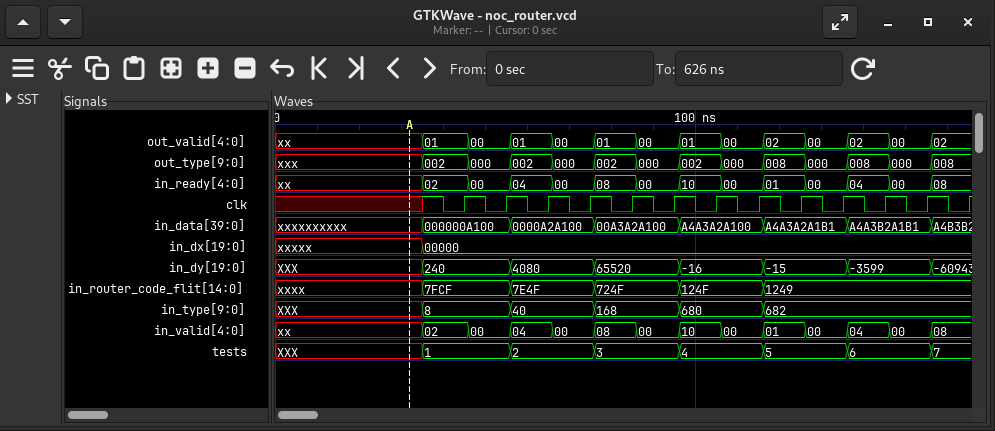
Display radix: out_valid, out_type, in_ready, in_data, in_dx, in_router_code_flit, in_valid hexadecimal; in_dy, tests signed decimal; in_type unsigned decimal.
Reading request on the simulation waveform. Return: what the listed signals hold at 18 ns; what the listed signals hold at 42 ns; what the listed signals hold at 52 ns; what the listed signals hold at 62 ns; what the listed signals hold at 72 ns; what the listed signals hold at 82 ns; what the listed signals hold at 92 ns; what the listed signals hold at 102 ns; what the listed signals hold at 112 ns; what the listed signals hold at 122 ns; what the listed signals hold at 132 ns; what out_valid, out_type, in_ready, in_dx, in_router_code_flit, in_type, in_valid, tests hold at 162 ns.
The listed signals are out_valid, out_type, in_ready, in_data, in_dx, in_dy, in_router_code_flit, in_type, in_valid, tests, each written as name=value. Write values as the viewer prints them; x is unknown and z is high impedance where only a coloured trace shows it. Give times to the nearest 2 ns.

out_valid=xx, out_type=xxx, in_ready=xx, in_data=xxxxxxxxxx, in_dx=xxxxx, in_dy=XXX, in_router_code_flit=xxxx, in_type=XXX, in_valid=xx, tests=XXX
out_valid=01, out_type=002, in_ready=02, in_data=000000A100, in_dx=00000, in_dy=240, in_router_code_flit=7FCF, in_type=8, in_valid=02, tests=1
out_valid=00, out_type=000, in_ready=00, in_data=000000A100, in_dx=00000, in_dy=240, in_router_code_flit=7FCF, in_type=8, in_valid=00, tests=1
out_valid=01, out_type=002, in_ready=04, in_data=0000A2A100, in_dx=00000, in_dy=4080, in_router_code_flit=7E4F, in_type=40, in_valid=04, tests=2
out_valid=00, out_type=000, in_ready=00, in_data=0000A2A100, in_dx=00000, in_dy=4080, in_router_code_flit=7E4F, in_type=40, in_valid=00, tests=2
out_valid=01, out_type=002, in_ready=08, in_data=00A3A2A100, in_dx=00000, in_dy=65520, in_router_code_flit=724F, in_type=168, in_valid=08, tests=3
out_valid=00, out_type=000, in_ready=00, in_data=00A3A2A100, in_dx=00000, in_dy=65520, in_router_code_flit=724F, in_type=168, in_valid=00, tests=3
out_valid=01, out_type=002, in_ready=10, in_data=A4A3A2A100, in_dx=00000, in_dy=-16, in_router_code_flit=124F, in_type=680, in_valid=10, tests=4
out_valid=00, out_type=000, in_ready=00, in_data=A4A3A2A100, in_dx=00000, in_dy=-16, in_router_code_flit=124F, in_type=680, in_valid=00, tests=4
out_valid=02, out_type=008, in_ready=01, in_data=A4A3A2A1B1, in_dx=00000, in_dy=-15, in_router_code_flit=1249, in_type=682, in_valid=01, tests=5
out_valid=00, out_type=000, in_ready=00, in_data=A4A3A2A1B1, in_dx=00000, in_dy=-15, in_router_code_flit=1249, in_type=682, in_valid=00, tests=5
out_valid=02, out_type=008, in_ready=08, in_dx=00000, in_router_code_flit=1249, in_type=682, in_valid=08, tests=7
